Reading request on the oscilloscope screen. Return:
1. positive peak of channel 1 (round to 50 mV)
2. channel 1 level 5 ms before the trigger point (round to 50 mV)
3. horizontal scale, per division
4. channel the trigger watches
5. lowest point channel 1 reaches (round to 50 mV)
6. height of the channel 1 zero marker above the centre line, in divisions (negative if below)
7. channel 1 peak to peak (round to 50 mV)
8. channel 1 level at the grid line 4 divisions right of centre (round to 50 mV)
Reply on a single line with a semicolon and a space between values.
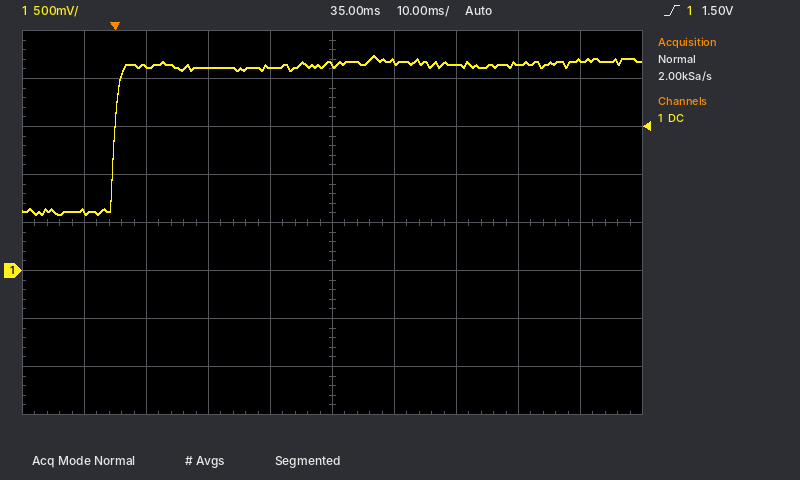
2.25 V; 600 mV; 10 ms; channel 1; 600 mV; -1.0 div; 1.65 V; 2.20 V
